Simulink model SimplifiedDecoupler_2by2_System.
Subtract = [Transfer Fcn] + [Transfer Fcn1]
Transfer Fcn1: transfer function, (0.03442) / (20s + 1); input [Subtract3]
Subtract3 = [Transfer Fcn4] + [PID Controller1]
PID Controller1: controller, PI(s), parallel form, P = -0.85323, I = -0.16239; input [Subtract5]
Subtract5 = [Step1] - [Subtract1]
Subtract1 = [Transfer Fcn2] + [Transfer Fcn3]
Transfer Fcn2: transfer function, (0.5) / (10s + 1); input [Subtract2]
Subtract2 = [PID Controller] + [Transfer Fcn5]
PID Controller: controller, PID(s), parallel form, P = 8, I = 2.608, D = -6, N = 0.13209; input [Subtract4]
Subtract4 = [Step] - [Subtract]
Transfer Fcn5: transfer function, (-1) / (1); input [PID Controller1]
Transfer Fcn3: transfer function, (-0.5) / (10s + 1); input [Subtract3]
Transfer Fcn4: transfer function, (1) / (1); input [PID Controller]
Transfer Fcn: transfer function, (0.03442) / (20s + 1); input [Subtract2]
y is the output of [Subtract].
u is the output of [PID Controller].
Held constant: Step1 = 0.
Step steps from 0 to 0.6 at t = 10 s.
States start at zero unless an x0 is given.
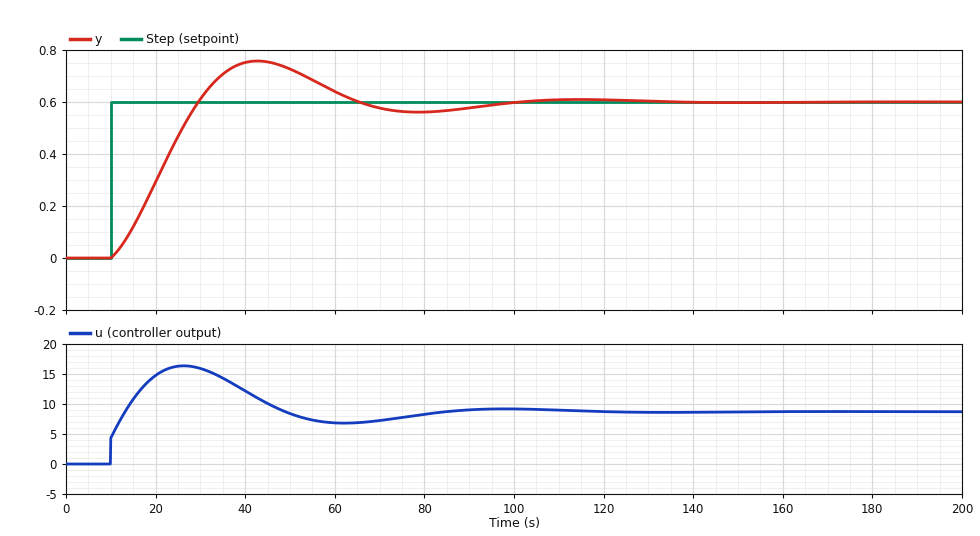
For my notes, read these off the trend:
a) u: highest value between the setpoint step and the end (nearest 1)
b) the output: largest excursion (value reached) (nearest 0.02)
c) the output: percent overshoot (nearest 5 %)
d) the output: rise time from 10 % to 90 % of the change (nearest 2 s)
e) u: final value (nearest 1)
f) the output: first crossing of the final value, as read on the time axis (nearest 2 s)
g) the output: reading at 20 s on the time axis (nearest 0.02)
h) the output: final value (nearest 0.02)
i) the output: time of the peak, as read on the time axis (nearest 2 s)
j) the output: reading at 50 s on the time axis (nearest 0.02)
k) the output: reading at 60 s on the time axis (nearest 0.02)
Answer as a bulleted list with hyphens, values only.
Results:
- 16
- 0.76
- 25 %
- 14 s
- 9
- 30 s
- 0.30
- 0.60
- 42 s
- 0.72
- 0.64
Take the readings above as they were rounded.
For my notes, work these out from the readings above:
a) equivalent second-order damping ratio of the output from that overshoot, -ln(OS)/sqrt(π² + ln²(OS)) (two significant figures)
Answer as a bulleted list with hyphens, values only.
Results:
- 0.40
